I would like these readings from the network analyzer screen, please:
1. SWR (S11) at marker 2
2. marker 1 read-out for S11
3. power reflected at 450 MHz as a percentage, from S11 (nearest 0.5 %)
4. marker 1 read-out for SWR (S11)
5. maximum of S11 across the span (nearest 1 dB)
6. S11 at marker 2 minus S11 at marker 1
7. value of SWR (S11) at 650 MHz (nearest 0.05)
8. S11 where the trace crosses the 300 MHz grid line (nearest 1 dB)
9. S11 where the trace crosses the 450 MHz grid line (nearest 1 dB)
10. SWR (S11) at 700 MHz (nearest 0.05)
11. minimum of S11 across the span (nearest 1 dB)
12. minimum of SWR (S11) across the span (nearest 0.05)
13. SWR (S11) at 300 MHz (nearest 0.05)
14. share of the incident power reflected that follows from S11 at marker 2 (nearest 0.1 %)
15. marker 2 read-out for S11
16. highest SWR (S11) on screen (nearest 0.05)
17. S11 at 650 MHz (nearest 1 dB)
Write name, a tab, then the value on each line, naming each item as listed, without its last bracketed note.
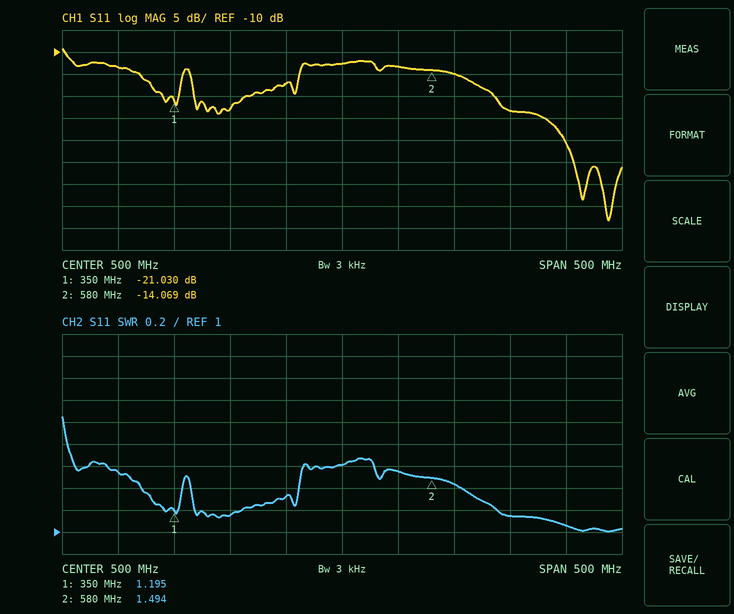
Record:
SWR (S11) at marker 2	1.494
marker 1 read-out for S11	-21.030 dB
power reflected at 450 MHz as a percentage, from S11	2.0 %
marker 1 read-out for SWR	1.195
maximum of S11 across the span	-9 dB
S11 at marker 2 minus S11 at marker 1	6.961 dB
value of SWR (S11) at 650 MHz	1.15
S11 where the trace crosses the 300 MHz grid line	-13 dB
S11 where the trace crosses the 450 MHz grid line	-17 dB
SWR (S11) at 700 MHz	1.05
minimum of S11 across the span	-48 dB
minimum of SWR (S11) across the span	1.00
SWR (S11) at 300 MHz	1.55
share of the incident power reflected that follows from S11 at marker 2	3.9 %
marker 2 read-out for S11	-14.069 dB
highest SWR (S11) on screen	2.05
S11 at 650 MHz	-23 dB
